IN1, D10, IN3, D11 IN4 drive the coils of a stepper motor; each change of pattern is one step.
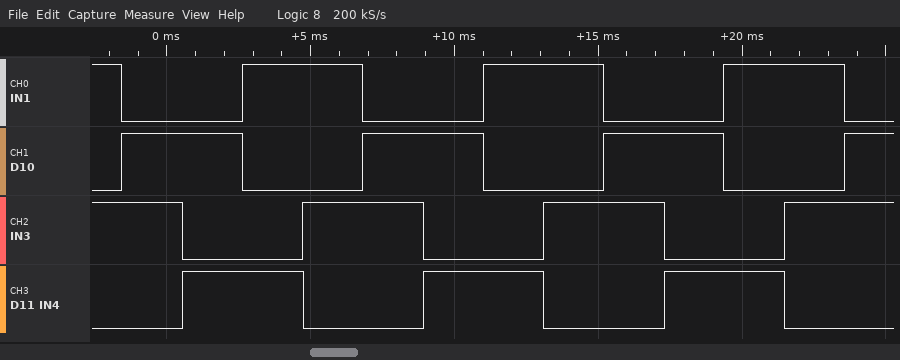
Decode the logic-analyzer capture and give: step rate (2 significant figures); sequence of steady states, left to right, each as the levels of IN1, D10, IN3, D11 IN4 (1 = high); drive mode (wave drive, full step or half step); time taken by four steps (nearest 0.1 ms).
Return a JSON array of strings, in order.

["480 steps/s", "1010 0110 0101 1001 1010 0110 0101 1001 1010 0110 0101 1001 1010 0110", "full step", "8.4 ms"]
